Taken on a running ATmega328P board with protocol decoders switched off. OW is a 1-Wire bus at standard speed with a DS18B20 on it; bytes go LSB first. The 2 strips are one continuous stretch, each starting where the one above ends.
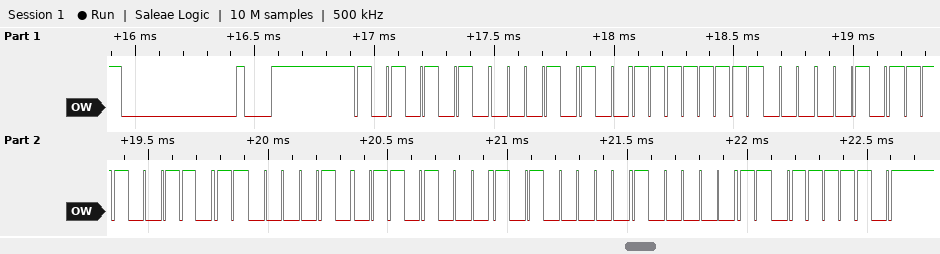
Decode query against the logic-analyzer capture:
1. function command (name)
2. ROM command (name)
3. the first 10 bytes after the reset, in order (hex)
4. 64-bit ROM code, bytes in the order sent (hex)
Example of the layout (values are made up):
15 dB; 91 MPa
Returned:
Read Scratchpad; Match ROM; 55 28 FF A0 67 43 16 05 C1 BE; 28 FF A0 67 43 16 05 C1
